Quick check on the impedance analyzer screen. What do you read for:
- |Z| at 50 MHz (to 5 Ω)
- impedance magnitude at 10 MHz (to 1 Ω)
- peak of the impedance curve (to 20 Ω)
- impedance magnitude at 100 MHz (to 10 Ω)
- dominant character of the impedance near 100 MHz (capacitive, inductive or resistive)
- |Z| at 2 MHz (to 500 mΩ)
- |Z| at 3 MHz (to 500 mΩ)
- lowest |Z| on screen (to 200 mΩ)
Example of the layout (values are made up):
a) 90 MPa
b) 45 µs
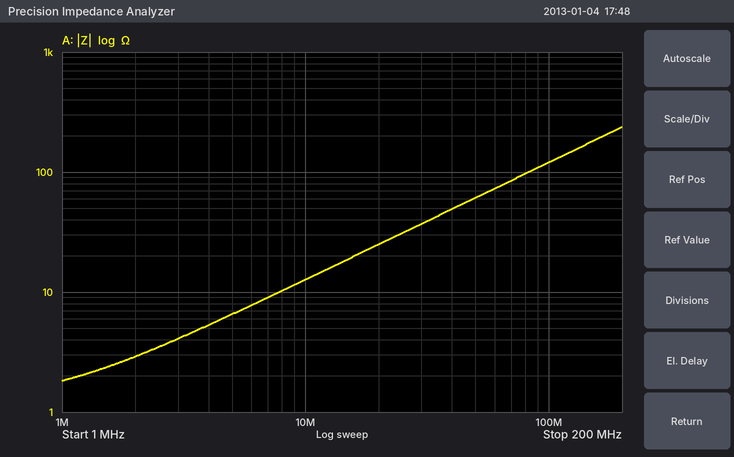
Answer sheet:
a) 60 Ω
b) 13 Ω
c) 240 Ω
d) 120 Ω
e) inductive
f) 3.0 Ω
g) 4.0 Ω
h) 1.8 Ω
